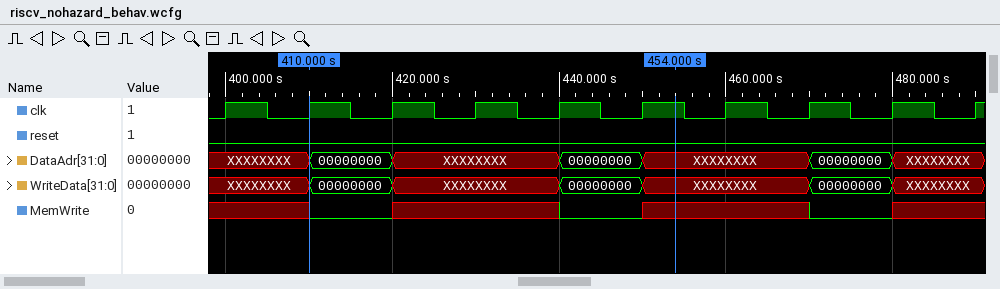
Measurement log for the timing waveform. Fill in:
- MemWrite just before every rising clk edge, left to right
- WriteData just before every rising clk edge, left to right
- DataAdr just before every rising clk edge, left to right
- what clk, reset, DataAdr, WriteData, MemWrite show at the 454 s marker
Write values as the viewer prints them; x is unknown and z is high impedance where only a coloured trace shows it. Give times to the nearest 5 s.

x x 0 x x 0 x x 0 x
XXXXXXXX, XXXXXXXX, 00000000, XXXXXXXX, XXXXXXXX, 00000000, XXXXXXXX, XXXXXXXX, 00000000, XXXXXXXX
XXXXXXXX, XXXXXXXX, 00000000, XXXXXXXX, XXXXXXXX, 00000000, XXXXXXXX, XXXXXXXX, 00000000, XXXXXXXX
clk=1, reset=0, DataAdr=XXXXXXXX, WriteData=XXXXXXXX, MemWrite=x
